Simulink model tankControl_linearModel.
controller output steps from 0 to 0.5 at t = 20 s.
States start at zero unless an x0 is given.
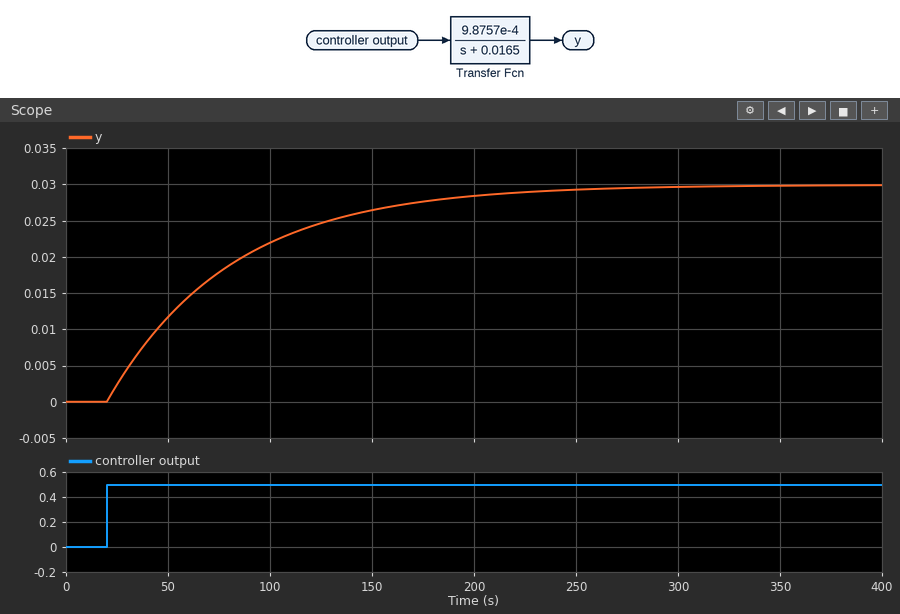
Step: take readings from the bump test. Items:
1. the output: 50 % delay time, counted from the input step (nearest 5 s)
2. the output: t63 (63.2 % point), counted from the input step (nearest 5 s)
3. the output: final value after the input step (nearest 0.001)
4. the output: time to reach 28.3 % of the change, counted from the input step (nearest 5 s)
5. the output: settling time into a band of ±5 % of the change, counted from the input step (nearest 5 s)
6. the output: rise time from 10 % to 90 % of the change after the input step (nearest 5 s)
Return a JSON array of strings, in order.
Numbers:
["40 s", "60 s", "0.030", "20 s", "180 s", "135 s"]
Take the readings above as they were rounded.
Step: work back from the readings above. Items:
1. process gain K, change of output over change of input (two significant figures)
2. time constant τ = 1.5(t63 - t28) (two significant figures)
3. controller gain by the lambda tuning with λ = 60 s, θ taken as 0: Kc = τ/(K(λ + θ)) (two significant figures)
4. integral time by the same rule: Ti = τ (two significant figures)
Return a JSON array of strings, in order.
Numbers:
["0.060", "60 s", "17", "60 s"]
